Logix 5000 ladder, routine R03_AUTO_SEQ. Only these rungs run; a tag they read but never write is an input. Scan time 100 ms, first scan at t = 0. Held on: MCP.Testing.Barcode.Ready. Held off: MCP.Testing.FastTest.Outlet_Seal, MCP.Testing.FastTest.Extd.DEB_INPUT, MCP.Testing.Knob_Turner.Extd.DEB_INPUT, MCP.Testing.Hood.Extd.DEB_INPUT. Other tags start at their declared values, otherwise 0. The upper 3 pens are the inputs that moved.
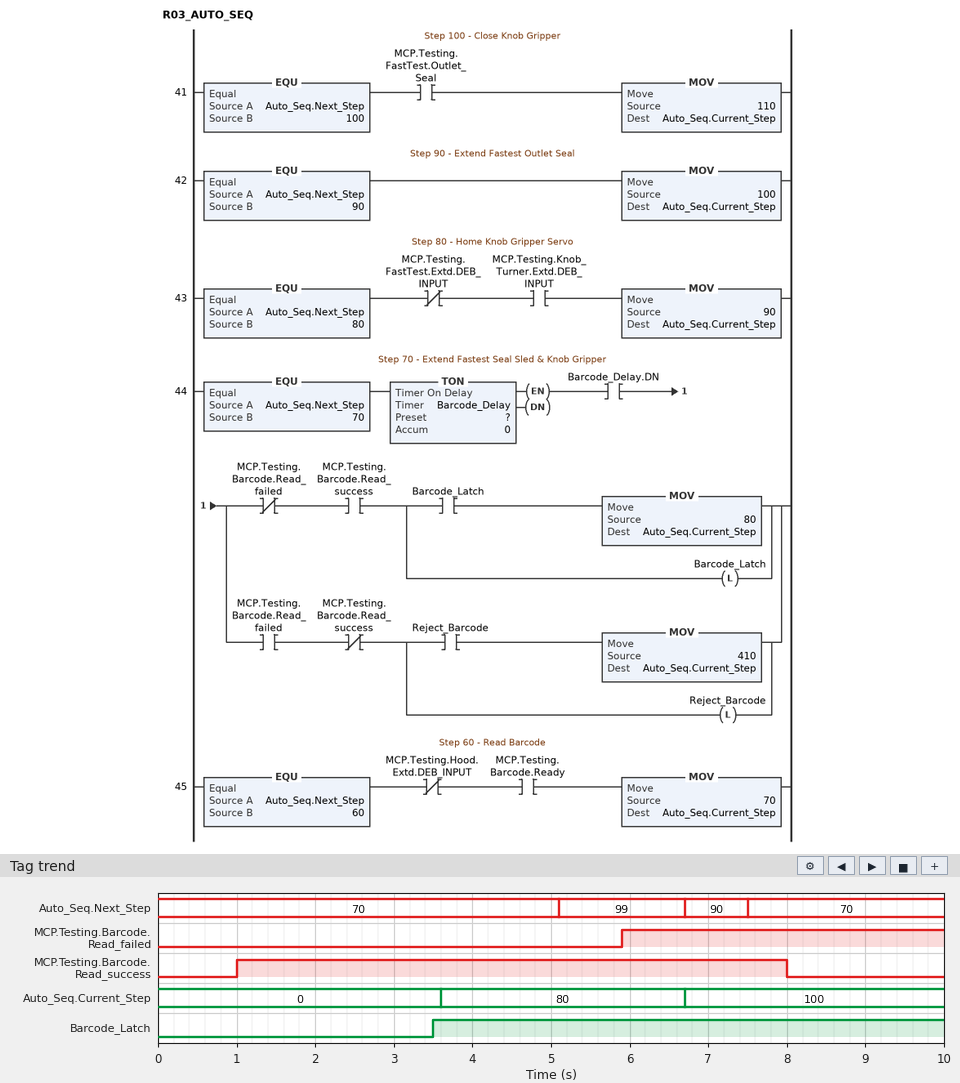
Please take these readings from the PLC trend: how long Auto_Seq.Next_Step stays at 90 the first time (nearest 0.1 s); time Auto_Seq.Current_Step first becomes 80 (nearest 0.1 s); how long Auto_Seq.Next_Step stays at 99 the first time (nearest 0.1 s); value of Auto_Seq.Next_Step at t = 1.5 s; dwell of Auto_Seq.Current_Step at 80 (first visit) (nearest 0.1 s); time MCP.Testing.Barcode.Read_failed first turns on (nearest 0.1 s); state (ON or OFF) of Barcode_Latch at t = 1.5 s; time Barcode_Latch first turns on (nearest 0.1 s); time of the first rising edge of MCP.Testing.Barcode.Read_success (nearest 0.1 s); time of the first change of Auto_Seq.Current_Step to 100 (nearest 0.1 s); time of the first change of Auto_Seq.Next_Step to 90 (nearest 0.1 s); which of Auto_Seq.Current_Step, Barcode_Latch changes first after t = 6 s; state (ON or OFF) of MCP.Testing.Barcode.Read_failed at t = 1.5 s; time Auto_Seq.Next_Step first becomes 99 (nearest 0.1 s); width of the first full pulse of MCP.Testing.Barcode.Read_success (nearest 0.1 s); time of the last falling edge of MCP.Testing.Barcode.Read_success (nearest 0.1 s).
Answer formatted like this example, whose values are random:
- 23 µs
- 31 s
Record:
- 0.8 s
- 3.6 s
- 1.6 s
- 70
- 3.1 s
- 5.9 s
- OFF
- 3.5 s
- 1.0 s
- 6.7 s
- 6.7 s
- Auto_Seq.Current_Step
- OFF
- 5.1 s
- 7.0 s
- 8.0 s
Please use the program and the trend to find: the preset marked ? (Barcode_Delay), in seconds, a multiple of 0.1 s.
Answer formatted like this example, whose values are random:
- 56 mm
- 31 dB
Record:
- 3.5 s
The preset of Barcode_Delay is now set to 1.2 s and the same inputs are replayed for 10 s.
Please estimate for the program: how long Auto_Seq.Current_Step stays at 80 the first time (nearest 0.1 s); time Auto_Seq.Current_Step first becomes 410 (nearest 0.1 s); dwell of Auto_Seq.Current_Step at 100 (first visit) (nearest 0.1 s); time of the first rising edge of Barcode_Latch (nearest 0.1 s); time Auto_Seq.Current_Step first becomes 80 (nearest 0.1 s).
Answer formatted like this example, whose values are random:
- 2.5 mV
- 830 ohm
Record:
- 5.4 s
- 8.8 s
- 2.1 s
- 1.2 s
- 1.3 s
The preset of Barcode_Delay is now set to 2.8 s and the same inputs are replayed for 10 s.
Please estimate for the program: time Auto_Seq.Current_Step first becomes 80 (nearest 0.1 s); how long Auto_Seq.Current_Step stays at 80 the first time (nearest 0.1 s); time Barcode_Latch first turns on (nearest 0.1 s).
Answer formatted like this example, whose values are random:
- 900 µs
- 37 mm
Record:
- 2.9 s
- 3.8 s
- 2.8 s
